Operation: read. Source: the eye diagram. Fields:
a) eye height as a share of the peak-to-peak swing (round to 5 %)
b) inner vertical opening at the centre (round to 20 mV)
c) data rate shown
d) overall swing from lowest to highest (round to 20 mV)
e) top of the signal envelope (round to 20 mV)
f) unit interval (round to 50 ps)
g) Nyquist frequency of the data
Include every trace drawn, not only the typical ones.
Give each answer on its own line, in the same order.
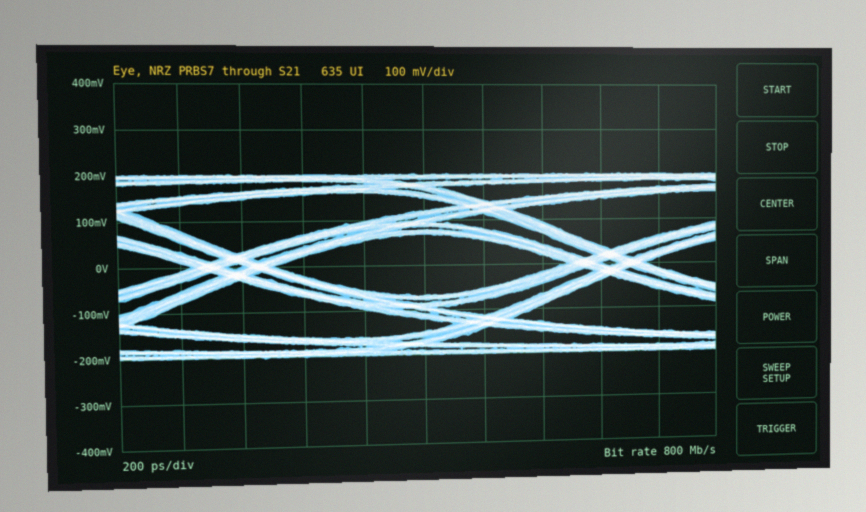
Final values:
35 %
140 mV
800 Mb/s
400 mV
200 mV
1.25 ns
400 MHz
